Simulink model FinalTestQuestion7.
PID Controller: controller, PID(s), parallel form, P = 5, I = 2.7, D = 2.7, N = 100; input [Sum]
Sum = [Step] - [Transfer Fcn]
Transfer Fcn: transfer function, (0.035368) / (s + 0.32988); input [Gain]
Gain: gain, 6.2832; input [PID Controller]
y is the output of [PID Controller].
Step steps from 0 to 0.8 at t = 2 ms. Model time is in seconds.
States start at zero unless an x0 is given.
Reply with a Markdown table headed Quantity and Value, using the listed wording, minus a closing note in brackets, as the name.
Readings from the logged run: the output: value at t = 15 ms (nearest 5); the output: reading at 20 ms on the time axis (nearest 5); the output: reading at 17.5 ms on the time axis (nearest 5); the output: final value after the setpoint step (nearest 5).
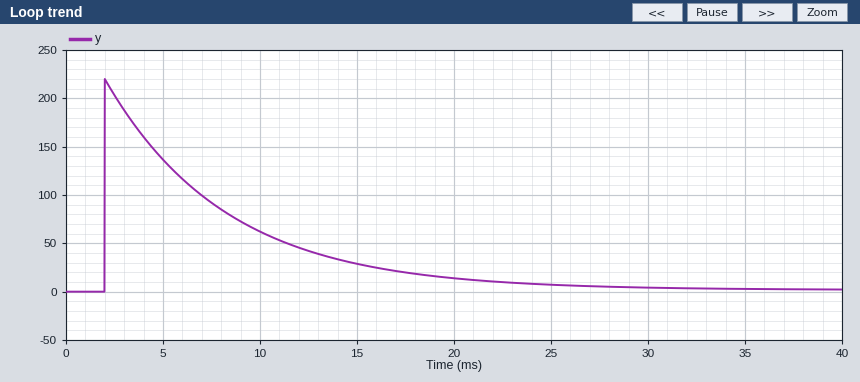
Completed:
| Quantity | Value |
|---|---|
| the output: value at t = 15 ms | 30 |
| the output: reading at 20 ms on the time axis | 15 |
| the output: reading at 17.5 ms on the time axis | 20 |
| the output: final value after the setpoint step | 0 |
